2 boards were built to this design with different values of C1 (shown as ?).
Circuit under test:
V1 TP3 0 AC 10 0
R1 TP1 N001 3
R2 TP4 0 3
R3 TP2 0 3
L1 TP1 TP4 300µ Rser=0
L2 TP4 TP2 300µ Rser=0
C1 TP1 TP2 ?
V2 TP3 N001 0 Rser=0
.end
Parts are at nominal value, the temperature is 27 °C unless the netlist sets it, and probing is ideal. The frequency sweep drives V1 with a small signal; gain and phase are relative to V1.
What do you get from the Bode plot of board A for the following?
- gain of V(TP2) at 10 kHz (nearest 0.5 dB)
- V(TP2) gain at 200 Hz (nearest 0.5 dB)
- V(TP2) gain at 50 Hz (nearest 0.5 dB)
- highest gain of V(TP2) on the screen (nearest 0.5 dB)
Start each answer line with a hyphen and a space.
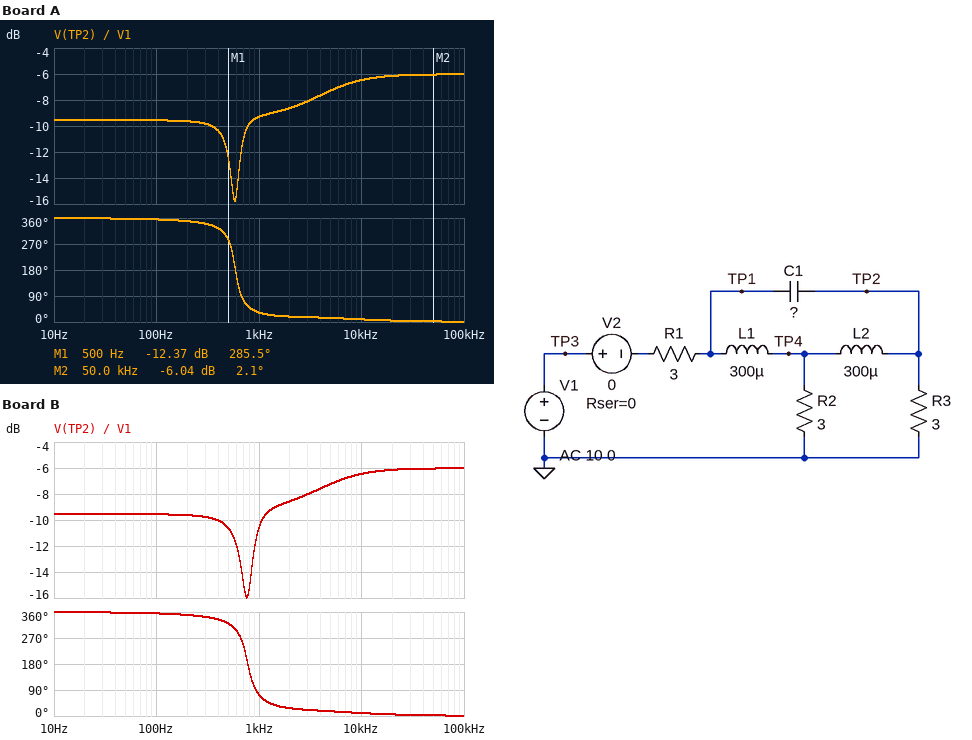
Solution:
- -6.5 dB
- -9.5 dB
- -9.5 dB
- -6.0 dB
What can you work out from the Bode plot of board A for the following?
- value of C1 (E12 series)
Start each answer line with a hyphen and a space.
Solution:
- 120 µF
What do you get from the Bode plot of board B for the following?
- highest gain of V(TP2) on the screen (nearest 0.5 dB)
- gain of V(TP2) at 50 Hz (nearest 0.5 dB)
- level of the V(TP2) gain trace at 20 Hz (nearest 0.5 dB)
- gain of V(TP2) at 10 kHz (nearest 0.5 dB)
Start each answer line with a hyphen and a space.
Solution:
- -6.0 dB
- -9.5 dB
- -9.5 dB
- -6.5 dB
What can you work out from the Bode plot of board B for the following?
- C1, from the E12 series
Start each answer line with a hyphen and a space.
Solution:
- 68 µF
